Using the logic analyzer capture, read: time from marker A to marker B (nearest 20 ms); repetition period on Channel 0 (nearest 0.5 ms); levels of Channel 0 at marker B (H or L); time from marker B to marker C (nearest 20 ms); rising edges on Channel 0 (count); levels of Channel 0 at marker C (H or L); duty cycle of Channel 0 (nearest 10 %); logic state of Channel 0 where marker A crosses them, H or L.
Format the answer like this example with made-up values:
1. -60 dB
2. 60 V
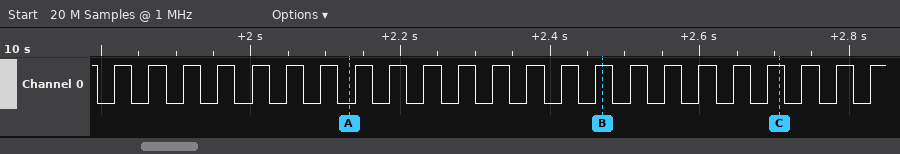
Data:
1. 340 ms
2. 46 ms
3. Channel 0=H
4. 240 ms
5. 23
6. Channel 0=H
7. 50 %
8. Channel 0=L
